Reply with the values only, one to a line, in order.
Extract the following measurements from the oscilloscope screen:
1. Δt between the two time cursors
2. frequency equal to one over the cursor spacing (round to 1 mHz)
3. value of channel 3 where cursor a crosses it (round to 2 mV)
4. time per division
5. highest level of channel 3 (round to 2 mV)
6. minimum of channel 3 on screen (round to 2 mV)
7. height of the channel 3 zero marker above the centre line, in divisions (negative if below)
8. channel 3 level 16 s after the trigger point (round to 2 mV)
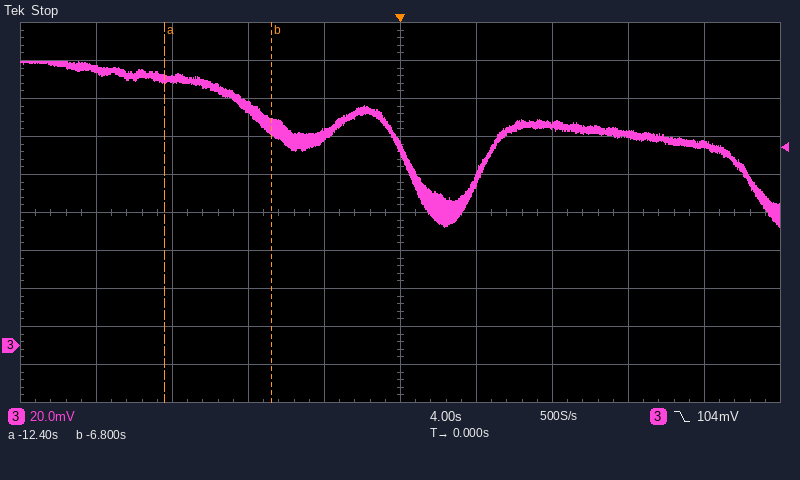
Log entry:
5.6 s
179 mHz
140 mV
4 s
150 mV
62 mV
-3.5 div
106 mV
